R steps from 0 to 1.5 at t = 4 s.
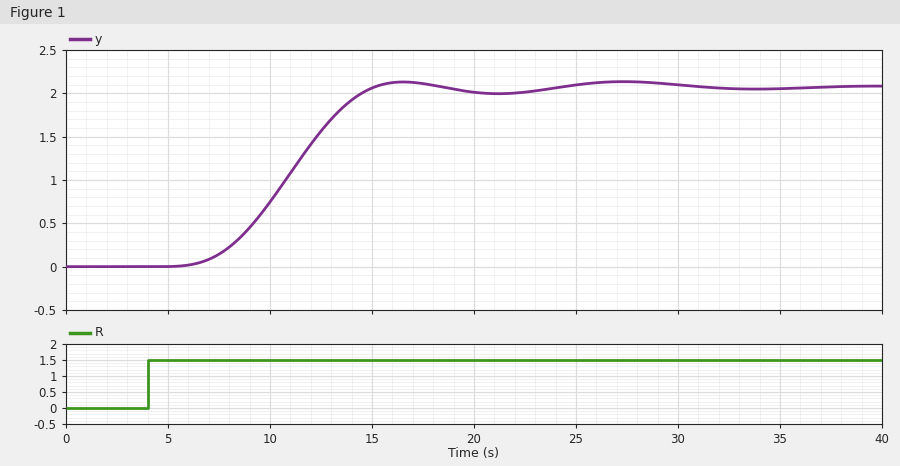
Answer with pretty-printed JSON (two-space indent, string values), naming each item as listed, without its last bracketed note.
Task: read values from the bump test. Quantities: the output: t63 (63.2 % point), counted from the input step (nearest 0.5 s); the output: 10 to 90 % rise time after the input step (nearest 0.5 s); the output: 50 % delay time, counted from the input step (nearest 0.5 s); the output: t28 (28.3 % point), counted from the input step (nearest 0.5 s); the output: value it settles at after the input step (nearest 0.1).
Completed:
{
  "the output: t63 (63.2 % point), counted from the input step": "7.5 s",
  "the output: 10 to 90 % rise time after the input step": "6.0 s",
  "the output: 50 % delay time, counted from the input step": "7.0 s",
  "the output: t28 (28.3 % point), counted from the input step": "5.5 s",
  "the output: value it settles at after the input step": "2.1"
}
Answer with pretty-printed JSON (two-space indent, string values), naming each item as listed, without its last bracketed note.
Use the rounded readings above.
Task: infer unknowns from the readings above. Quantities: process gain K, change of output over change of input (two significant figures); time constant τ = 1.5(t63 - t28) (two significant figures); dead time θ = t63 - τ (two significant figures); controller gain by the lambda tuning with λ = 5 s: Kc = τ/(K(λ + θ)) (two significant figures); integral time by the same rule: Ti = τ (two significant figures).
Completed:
{
  "process gain K, change of output over change of input": "1.4",
  "time constant τ = 1.5(t63 - t28)": "3.0 s",
  "dead time θ = t63 - τ": "4.5 s",
  "controller gain by the lambda tuning with λ = 5 s: Kc = τ/(K(λ + θ))": "0.23",
  "integral time by the same rule: Ti = τ": "3.0 s"
}
